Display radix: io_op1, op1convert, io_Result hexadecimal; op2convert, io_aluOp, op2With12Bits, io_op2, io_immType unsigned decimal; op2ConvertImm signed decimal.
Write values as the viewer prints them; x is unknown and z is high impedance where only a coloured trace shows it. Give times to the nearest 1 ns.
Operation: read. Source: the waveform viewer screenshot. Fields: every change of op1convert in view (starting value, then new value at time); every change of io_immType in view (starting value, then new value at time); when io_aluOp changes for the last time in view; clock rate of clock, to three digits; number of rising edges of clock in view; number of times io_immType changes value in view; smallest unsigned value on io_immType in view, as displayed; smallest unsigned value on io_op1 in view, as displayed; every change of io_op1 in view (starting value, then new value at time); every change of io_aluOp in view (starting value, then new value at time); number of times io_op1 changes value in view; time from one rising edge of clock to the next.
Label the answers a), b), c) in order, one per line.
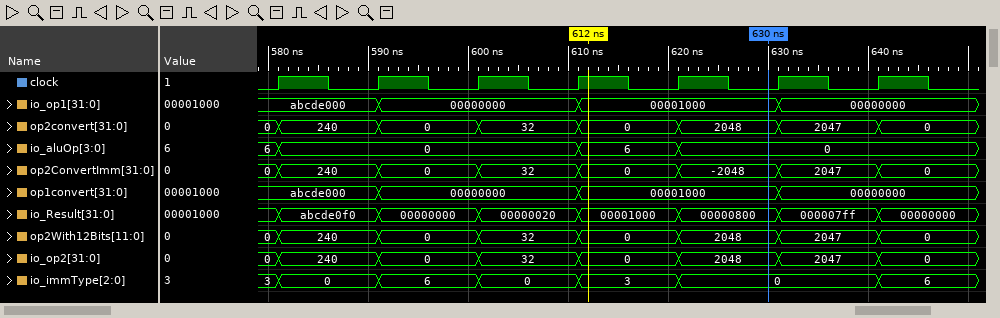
a) abcde000, 00000000 at 591 ns, 00001000 at 611 ns, 00000000 at 631 ns
b) 3, 0 at 581 ns, 6 at 591 ns, 0 at 601 ns, 3 at 611 ns, 0 at 621 ns, 6 at 641 ns
c) 621 ns
d) 100 MHz
e) 7
f) 6
g) 0
h) 00000000
i) abcde000, 00000000 at 591 ns, 00001000 at 611 ns, 00000000 at 631 ns
j) 6, 0 at 581 ns, 6 at 611 ns, 0 at 621 ns
k) 3
l) 10 ns
